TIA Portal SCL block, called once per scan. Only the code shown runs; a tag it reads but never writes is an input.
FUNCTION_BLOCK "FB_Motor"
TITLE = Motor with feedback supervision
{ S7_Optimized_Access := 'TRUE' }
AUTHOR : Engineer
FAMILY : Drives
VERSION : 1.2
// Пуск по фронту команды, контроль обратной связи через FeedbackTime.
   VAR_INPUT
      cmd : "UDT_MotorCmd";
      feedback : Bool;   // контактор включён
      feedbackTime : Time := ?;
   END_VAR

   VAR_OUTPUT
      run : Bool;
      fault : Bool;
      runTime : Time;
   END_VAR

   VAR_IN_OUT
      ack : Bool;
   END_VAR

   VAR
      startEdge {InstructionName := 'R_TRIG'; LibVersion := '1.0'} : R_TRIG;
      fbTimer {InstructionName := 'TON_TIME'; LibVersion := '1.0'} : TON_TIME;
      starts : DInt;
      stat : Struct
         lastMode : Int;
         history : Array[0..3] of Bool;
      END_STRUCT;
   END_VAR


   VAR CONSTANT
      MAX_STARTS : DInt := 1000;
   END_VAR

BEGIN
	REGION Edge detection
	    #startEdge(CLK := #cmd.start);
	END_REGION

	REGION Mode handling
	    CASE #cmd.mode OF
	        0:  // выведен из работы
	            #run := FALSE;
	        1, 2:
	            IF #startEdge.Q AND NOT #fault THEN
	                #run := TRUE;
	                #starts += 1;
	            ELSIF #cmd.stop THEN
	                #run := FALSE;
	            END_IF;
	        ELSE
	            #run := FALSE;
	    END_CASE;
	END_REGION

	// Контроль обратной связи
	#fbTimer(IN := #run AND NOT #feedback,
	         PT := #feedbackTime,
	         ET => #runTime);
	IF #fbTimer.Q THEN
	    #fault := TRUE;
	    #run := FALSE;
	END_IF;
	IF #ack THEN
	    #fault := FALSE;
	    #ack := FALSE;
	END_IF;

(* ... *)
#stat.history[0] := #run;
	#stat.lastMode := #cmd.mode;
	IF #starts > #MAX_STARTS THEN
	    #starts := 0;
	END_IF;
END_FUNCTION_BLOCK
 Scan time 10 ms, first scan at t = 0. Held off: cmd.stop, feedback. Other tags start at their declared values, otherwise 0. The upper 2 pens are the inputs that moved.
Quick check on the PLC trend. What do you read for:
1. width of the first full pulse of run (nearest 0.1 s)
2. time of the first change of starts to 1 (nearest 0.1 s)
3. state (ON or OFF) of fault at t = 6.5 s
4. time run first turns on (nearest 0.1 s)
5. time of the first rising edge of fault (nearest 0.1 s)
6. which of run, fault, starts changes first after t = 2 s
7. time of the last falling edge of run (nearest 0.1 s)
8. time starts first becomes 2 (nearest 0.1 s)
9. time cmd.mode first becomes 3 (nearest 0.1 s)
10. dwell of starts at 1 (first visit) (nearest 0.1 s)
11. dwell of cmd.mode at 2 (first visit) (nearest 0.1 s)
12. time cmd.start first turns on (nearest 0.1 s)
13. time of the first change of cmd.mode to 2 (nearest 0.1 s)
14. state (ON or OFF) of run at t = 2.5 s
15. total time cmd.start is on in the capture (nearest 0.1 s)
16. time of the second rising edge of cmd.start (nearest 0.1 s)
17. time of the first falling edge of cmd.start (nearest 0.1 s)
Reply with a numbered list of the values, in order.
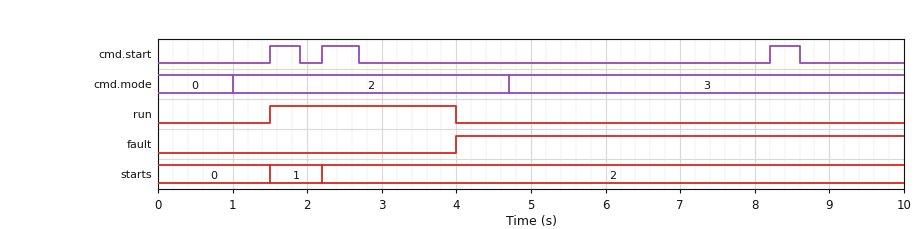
1. 2.5 s
2. 1.5 s
3. ON
4. 1.5 s
5. 4.0 s
6. starts
7. 4.0 s
8. 2.2 s
9. 4.7 s
10. 0.7 s
11. 3.7 s
12. 1.5 s
13. 1.0 s
14. ON
15. 1.3 s
16. 2.2 s
17. 1.9 s
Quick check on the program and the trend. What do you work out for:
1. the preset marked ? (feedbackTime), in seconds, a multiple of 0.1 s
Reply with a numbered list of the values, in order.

1. 2.5 s
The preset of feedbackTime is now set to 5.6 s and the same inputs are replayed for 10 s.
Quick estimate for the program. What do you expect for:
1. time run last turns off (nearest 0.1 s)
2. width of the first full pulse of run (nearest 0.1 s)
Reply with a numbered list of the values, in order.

1. 4.7 s
2. 3.2 s
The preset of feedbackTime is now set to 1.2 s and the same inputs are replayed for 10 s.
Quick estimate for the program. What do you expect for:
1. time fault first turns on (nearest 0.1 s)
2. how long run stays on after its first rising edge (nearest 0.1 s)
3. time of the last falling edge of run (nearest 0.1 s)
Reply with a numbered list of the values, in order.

1. 2.7 s
2. 1.2 s
3. 2.7 s
